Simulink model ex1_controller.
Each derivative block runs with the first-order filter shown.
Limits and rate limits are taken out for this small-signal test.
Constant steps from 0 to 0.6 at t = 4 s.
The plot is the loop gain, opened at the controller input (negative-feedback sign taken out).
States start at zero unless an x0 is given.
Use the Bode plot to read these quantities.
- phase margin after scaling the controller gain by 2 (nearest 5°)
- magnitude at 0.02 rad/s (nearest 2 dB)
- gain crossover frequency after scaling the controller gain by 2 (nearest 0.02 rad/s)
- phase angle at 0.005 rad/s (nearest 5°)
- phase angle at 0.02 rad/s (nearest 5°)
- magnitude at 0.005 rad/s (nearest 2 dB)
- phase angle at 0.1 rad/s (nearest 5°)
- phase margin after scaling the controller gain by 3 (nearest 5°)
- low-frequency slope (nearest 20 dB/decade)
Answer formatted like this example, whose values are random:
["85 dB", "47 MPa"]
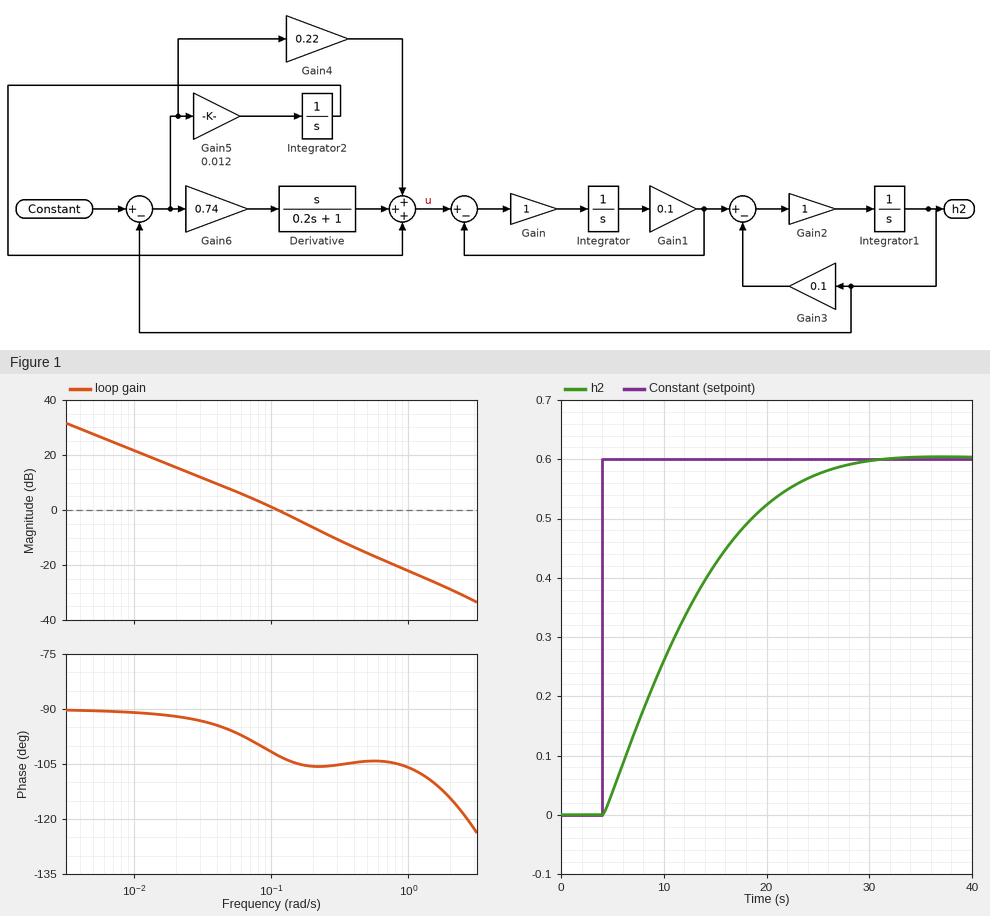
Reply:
["75°", "16 dB", "0.20 rad/s", "-90°", "-90°", "28 dB", "-100°", "75°", "-20 dB/decade"]
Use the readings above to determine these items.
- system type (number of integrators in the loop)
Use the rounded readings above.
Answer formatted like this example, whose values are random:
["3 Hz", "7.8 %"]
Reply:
["1"]
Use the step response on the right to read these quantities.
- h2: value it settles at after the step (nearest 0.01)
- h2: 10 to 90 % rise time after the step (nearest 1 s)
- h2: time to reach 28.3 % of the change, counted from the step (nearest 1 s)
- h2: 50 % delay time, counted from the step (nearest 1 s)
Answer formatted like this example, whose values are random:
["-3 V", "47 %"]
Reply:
["0.60", "16 s", "4 s", "7 s"]
